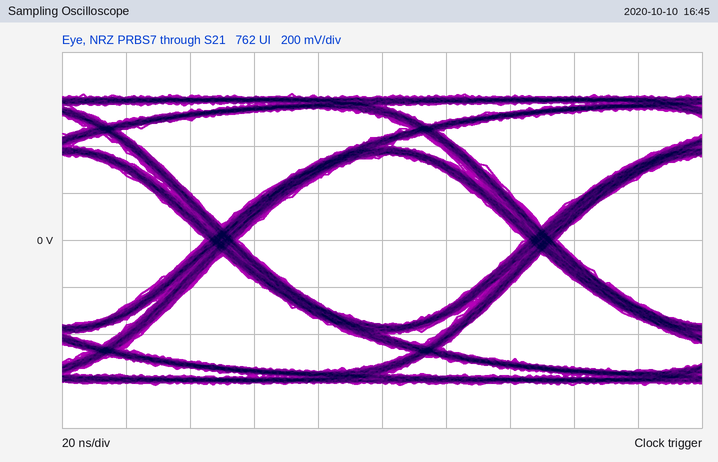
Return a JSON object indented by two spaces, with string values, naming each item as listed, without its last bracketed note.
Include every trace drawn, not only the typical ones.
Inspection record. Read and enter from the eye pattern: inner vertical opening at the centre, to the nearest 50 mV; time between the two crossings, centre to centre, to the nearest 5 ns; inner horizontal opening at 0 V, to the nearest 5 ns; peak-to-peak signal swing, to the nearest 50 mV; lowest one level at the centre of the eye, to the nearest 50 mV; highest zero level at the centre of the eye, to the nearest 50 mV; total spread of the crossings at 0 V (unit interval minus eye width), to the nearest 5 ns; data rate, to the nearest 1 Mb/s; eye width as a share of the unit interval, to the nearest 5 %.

{
  "inner vertical opening at the centre, to the nearest 50 mV": "700 mV",
  "time between the two crossings, centre to centre, to the nearest 5 ns": "100 ns",
  "inner horizontal opening at 0 V, to the nearest 5 ns": "90 ns",
  "peak-to-peak signal swing, to the nearest 50 mV": "1.25 V",
  "lowest one level at the centre of the eye, to the nearest 50 mV": "350 mV",
  "highest zero level at the centre of the eye, to the nearest 50 mV": "-350 mV",
  "total spread of the crossings at 0 V (unit interval minus eye width), to the nearest 5 ns": "10 ns",
  "data rate, to the nearest 1 Mb/s": "10 Mb/s",
  "eye width as a share of the unit interval, to the nearest 5 %": "90 %"
}
